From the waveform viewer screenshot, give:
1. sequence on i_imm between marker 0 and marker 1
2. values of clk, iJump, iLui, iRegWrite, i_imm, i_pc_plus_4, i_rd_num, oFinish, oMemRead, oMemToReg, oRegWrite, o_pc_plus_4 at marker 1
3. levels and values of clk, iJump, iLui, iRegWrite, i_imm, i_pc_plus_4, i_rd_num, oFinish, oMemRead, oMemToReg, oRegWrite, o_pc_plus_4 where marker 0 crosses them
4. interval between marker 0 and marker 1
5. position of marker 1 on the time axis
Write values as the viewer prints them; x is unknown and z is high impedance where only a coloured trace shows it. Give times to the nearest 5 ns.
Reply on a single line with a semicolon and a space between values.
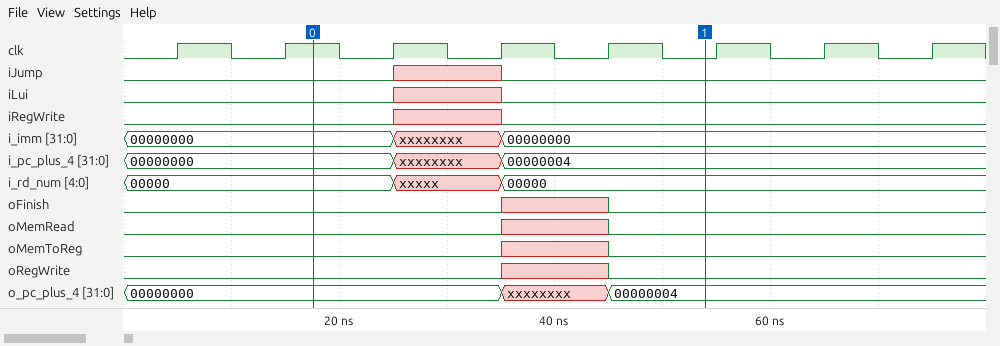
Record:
00000000, xxxxxxxx, 00000000; clk=0, iJump=0, iLui=0, iRegWrite=0, i_imm=00000000, i_pc_plus_4=00000004, i_rd_num=00000, oFinish=0, oMemRead=0, oMemToReg=0, oRegWrite=0, o_pc_plus_4=00000004; clk=1, iJump=0, iLui=0, iRegWrite=0, i_imm=00000000, i_pc_plus_4=00000000, i_rd_num=00000, oFinish=0, oMemRead=0, oMemToReg=0, oRegWrite=0, o_pc_plus_4=00000000; 35 ns; 55 ns
